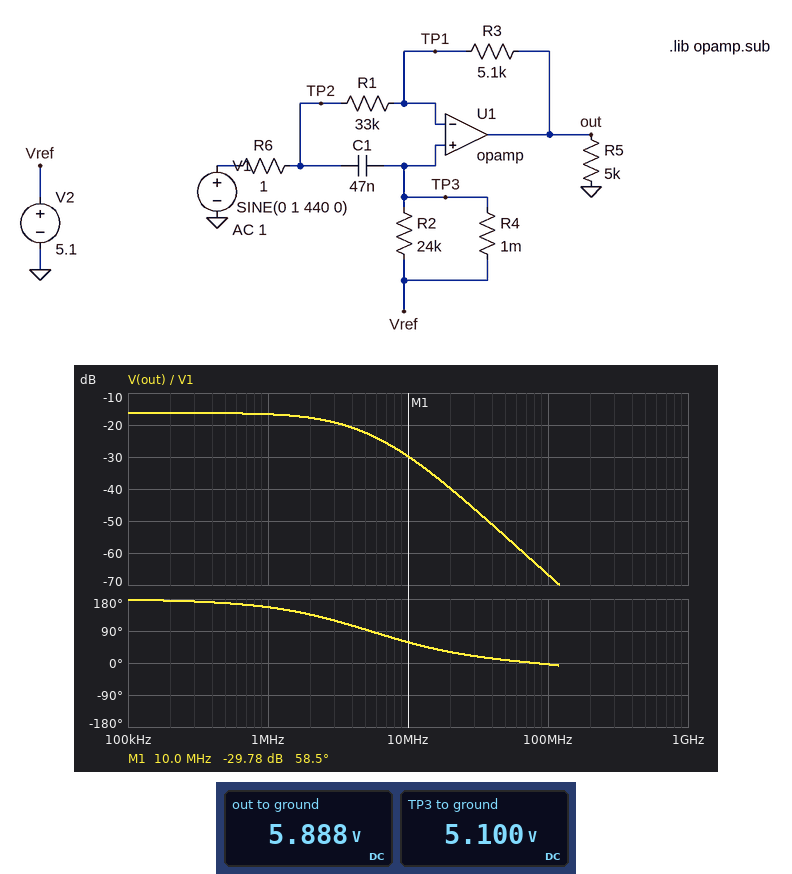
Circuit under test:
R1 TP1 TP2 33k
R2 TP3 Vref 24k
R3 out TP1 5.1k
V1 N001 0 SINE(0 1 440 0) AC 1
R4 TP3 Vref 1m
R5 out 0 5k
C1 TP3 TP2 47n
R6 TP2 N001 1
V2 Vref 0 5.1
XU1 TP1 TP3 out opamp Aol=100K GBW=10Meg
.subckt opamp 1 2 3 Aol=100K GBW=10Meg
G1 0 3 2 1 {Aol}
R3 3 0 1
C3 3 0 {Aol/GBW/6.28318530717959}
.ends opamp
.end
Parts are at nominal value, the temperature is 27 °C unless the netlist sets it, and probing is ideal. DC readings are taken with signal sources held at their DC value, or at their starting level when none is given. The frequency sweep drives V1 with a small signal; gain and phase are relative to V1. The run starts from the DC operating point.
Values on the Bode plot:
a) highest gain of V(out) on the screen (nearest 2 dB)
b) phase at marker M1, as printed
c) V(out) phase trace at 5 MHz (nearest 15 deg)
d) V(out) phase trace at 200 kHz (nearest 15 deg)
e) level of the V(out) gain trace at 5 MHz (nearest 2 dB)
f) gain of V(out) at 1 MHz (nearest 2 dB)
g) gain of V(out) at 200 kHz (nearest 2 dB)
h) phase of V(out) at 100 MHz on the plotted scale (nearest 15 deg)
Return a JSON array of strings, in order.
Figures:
["-16 dB", "58.5 deg", "90 deg", "180 deg", "-22 dB", "-16 dB", "-16 dB", "0 deg"]
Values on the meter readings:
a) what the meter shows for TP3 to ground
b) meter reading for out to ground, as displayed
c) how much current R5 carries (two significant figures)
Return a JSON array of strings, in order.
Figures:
["5.100 V", "5.888 V", "1.2 mA"]
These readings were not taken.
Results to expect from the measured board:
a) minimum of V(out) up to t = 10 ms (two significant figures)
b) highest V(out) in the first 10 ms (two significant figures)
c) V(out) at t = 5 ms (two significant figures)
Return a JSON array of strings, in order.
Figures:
["5.7 V", "6.0 V", "5.7 V"]
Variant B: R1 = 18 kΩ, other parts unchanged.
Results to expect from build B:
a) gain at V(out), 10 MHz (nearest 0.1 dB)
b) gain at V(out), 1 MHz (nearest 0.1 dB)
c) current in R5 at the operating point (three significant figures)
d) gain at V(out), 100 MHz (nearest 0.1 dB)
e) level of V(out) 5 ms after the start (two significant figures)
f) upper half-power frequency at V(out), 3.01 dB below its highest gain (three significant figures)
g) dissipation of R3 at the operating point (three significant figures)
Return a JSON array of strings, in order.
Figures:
["-25.1 dB", "-11.4 dB", "1.31 mA", "-62.5 dB", "6.3 V", "2.93 MHz", "409 µW"]
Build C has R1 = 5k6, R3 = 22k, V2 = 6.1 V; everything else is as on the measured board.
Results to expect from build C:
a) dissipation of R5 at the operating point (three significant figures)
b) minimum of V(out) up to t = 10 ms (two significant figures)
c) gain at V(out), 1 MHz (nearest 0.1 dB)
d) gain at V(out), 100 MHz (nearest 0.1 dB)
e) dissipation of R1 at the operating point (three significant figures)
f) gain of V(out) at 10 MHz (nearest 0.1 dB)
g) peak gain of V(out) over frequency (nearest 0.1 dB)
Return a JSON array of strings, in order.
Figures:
["181 mW", "26 V", "10.6 dB", "-51.4 dB", "6.64 mW", "-12.0 dB", "11.9 dB"]
